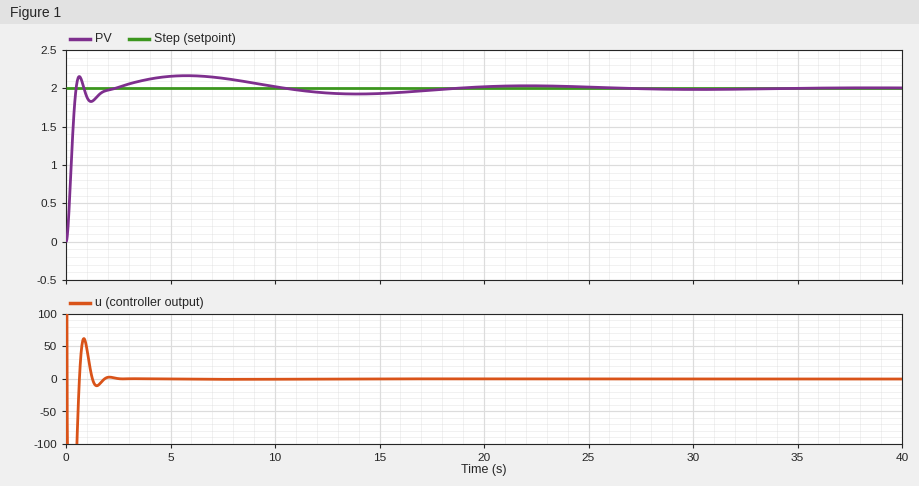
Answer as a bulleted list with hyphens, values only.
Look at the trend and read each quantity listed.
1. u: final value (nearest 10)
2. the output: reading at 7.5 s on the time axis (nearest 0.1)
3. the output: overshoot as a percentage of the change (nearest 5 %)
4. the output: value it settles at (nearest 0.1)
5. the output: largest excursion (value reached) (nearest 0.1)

- 0
- 2.1
- 10 %
- 2.0
- 2.2
